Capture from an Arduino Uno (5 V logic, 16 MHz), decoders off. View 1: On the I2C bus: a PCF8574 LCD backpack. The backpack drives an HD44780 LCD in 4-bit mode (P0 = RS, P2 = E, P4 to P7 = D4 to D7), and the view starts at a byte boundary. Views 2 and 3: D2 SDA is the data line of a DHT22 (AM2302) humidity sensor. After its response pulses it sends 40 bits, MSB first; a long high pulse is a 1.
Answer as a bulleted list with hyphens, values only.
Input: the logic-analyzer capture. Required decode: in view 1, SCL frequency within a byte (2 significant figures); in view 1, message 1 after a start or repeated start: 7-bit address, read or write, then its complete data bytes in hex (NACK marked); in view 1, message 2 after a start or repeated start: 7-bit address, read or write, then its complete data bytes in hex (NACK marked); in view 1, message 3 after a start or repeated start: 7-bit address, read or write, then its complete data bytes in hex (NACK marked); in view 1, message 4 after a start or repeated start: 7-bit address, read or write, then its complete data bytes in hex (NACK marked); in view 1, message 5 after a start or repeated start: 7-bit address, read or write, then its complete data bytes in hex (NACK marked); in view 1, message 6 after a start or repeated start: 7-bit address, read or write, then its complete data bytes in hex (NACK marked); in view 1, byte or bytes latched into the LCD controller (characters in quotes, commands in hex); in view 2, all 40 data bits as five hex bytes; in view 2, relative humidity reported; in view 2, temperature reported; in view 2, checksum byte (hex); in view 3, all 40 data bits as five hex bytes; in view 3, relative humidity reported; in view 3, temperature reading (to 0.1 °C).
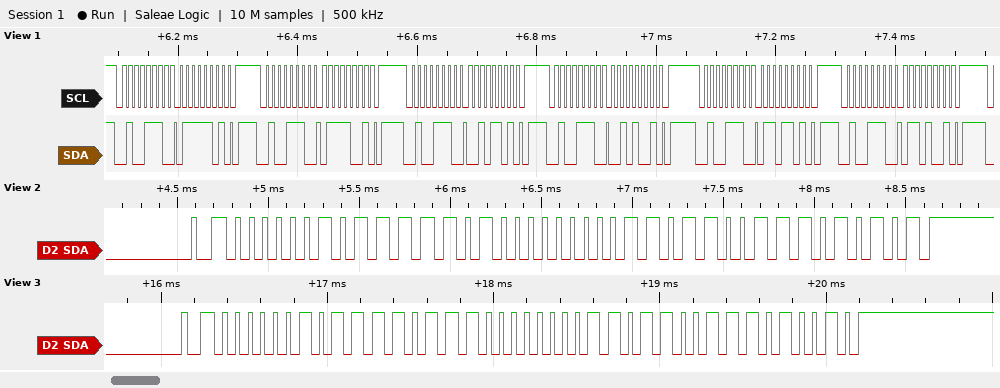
- 100 kHz
- 0x27 write: 7D
- 0x27 write: 79
- 0x27 write: 2D
- 0x27 write: 29
- 0x27 write: 6D
- 0x27 write: 69
- 'r'
- 02 FA 00 D9 D5
- 76.2 %
- 21.7 °C
- 0xD5
- 02 F7 00 D9 D2
- 75.9 %
- 21.7 °C
